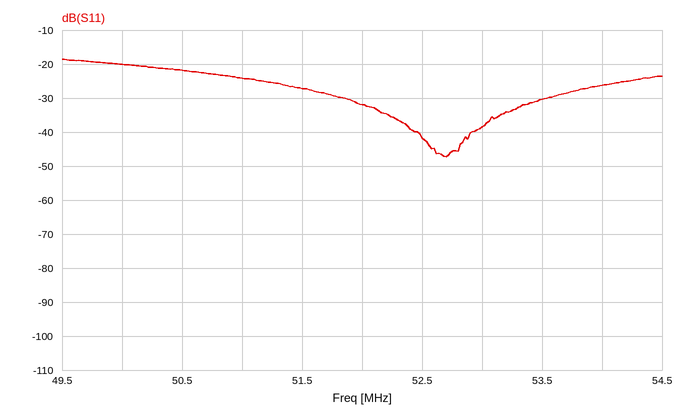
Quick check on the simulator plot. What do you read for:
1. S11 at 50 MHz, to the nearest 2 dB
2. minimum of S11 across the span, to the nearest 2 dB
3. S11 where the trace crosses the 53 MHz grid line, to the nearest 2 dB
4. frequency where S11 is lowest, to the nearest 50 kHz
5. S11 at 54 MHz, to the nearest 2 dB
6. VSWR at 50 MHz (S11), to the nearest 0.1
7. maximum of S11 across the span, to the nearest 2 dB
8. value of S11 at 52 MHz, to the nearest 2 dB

-20 dB
-48 dB
-38 dB
52.70 MHz
-26 dB
1.2
-18 dB
-32 dB
